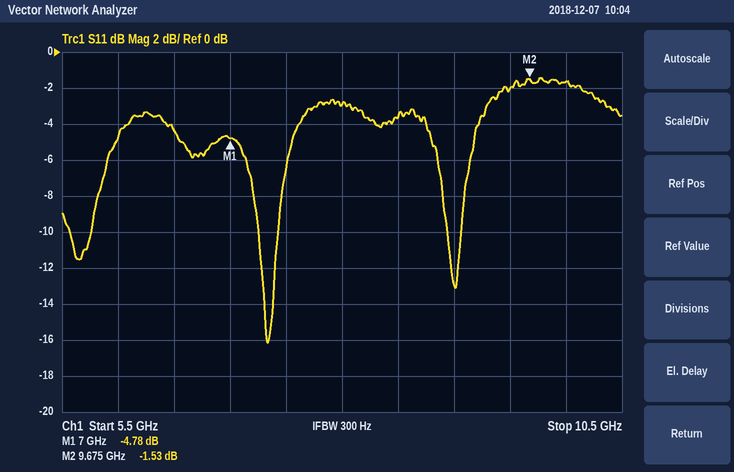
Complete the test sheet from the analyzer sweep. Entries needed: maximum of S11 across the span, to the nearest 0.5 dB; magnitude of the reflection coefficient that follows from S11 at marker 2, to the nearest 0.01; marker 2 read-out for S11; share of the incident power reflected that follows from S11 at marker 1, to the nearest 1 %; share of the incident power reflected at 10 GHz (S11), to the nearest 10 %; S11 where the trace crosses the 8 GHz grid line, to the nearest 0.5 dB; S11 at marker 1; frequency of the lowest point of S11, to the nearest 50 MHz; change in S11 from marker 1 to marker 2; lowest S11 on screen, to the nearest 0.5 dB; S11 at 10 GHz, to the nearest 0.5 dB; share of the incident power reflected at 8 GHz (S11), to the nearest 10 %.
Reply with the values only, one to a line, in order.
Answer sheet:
-1.5 dB
0.84
-1.53 dB
33 %
70 %
-3.0 dB
-4.78 dB
7.35 GHz
3.25 dB
-16.0 dB
-1.5 dB
50 %
